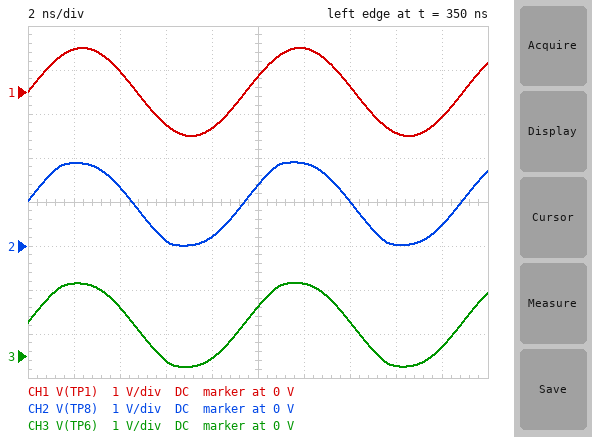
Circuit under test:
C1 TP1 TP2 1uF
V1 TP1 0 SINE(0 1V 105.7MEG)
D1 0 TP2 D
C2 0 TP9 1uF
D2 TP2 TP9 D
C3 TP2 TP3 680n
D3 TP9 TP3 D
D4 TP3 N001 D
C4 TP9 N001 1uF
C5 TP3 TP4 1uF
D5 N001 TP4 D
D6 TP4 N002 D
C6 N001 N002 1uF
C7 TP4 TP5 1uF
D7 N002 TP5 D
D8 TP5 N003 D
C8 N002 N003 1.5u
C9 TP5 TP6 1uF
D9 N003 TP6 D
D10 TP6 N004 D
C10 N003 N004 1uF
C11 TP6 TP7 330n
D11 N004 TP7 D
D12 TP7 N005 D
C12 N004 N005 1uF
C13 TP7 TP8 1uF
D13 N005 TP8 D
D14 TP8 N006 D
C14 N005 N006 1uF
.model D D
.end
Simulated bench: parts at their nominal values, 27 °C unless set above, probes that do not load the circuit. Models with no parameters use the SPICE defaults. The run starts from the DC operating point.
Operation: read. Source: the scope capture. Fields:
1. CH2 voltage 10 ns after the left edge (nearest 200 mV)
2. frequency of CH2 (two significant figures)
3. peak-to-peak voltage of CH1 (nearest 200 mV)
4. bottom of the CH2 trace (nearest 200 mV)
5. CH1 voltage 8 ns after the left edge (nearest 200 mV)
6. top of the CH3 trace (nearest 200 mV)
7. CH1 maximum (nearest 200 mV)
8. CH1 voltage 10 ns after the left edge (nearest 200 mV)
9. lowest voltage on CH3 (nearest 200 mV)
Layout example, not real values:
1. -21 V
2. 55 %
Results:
1. 1.4 V
2. 110 MHz
3. 2.0 V
4. 0 V
5. -800 mV
6. 1.6 V
7. 1.0 V
8. 400 mV
9. -200 mV
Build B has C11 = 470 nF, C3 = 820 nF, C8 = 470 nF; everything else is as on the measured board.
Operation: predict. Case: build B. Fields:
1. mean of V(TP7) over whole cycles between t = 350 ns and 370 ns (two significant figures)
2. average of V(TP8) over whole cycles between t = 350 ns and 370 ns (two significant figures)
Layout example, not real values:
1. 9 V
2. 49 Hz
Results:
1. 880 mV
2. 990 mV
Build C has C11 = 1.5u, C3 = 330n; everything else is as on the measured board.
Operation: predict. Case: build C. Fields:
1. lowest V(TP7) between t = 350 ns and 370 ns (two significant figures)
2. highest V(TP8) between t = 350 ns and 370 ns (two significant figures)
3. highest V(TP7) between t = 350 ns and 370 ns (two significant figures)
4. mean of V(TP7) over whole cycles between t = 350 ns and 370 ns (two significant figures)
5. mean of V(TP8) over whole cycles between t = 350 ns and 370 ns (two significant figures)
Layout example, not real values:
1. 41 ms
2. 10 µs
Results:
1. -210 mV
2. 1.8 V
3. 1.7 V
4. 730 mV
5. 830 mV
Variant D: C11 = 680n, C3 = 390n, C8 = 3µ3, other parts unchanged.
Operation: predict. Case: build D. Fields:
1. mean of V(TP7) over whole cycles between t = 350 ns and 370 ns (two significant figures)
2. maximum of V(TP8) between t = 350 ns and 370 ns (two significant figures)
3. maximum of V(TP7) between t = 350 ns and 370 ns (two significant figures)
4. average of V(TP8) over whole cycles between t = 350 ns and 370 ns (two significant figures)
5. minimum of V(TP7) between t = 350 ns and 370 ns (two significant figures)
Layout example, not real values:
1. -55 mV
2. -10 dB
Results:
1. 740 mV
2. 1.8 V
3. 1.7 V
4. 840 mV
5. -200 mV
